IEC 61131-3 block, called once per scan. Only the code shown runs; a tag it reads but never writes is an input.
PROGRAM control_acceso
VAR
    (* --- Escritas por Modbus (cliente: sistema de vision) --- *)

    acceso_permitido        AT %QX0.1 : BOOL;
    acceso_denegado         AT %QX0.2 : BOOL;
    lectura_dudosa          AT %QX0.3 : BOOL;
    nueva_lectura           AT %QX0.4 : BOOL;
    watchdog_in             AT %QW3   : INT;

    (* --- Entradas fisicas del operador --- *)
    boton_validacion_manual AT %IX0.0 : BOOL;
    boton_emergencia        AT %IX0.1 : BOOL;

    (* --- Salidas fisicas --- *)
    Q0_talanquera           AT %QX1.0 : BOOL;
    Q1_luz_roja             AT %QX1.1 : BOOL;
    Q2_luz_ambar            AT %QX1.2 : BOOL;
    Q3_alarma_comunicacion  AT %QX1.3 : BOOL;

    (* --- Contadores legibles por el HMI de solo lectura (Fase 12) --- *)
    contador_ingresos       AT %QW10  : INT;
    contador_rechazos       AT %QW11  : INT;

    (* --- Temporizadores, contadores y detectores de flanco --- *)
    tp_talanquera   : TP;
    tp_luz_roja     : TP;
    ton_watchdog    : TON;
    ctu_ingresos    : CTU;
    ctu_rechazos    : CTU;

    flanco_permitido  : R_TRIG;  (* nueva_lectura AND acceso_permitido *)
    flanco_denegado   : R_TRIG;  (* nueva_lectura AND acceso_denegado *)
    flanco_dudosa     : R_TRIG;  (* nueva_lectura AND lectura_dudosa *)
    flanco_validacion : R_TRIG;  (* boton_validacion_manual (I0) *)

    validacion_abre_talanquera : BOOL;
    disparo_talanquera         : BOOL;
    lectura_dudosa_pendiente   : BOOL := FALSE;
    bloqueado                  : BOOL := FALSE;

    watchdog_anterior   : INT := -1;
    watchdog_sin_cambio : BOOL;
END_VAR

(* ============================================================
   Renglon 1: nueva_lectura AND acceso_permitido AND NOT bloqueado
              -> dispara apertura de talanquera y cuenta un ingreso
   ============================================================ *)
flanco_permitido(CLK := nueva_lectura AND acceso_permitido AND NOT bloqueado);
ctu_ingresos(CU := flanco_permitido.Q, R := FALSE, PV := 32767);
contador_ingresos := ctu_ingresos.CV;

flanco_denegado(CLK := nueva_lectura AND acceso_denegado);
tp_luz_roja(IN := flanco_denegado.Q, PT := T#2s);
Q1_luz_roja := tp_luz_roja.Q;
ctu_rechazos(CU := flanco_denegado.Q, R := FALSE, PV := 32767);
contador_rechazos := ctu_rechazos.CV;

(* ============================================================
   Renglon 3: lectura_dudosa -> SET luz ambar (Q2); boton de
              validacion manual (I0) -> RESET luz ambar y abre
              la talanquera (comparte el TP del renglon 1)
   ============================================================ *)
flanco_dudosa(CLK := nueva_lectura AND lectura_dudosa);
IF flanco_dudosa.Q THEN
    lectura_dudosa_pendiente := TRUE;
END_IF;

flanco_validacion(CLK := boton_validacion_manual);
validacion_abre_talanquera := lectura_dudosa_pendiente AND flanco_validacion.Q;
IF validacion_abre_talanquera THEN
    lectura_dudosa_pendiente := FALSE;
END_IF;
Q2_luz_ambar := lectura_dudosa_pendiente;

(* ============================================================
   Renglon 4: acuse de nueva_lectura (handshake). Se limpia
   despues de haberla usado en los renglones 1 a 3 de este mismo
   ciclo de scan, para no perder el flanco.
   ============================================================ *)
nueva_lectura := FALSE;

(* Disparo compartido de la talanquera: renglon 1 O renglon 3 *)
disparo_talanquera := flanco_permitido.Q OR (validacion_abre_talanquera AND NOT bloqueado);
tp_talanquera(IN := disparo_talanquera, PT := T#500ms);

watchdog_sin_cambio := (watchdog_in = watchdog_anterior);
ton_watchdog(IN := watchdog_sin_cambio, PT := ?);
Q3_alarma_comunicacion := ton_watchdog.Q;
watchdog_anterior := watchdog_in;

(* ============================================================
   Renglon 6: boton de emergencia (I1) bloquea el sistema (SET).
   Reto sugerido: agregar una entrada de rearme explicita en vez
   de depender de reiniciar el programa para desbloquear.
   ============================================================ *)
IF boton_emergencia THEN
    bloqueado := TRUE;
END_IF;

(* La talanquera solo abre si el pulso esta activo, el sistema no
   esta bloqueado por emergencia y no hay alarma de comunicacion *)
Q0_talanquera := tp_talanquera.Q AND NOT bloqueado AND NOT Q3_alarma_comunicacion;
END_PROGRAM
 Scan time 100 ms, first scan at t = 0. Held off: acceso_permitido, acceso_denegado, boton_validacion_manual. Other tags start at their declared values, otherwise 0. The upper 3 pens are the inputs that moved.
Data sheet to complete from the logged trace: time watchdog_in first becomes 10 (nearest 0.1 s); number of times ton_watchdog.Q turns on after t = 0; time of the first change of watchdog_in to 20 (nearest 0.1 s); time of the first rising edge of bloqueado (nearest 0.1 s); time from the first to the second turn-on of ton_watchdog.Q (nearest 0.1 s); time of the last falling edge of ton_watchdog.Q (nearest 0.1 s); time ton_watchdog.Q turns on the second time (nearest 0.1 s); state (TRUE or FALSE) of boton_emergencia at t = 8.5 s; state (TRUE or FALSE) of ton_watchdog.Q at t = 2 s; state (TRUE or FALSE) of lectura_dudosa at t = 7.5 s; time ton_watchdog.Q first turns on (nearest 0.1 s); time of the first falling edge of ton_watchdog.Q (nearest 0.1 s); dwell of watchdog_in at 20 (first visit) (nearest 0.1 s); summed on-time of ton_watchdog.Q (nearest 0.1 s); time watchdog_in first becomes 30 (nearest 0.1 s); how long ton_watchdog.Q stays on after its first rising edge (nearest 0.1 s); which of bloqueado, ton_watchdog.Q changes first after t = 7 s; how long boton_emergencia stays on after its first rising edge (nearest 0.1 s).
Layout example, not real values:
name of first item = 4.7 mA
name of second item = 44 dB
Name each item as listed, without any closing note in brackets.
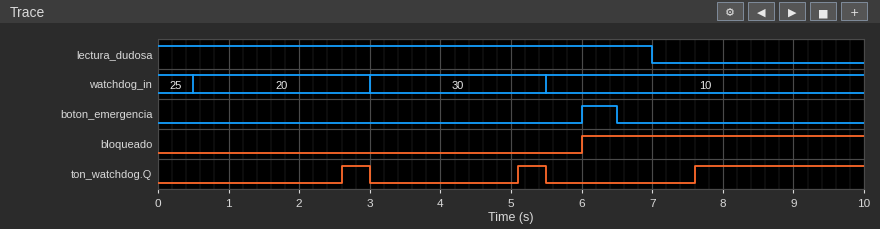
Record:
time watchdog_in first becomes 10 = 5.5 s
number of times ton_watchdog.Q turns on after t = 0 = 3
time of the first change of watchdog_in to 20 = 0.5 s
time of the first rising edge of bloqueado = 6.0 s
time from the first to the second turn-on of ton_watchdog.Q = 2.5 s
time of the last falling edge of ton_watchdog.Q = 5.5 s
time ton_watchdog.Q turns on the second time = 5.1 s
state (TRUE or FALSE) of boton_emergencia at t = 8.5 s = FALSE
state (TRUE or FALSE) of ton_watchdog.Q at t = 2 s = FALSE
state (TRUE or FALSE) of lectura_dudosa at t = 7.5 s = FALSE
time ton_watchdog.Q first turns on = 2.6 s
time of the first falling edge of ton_watchdog.Q = 3.0 s
dwell of watchdog_in at 20 (first visit) = 2.5 s
summed on-time of ton_watchdog.Q = 3.2 s
time watchdog_in first becomes 30 = 3.0 s
how long ton_watchdog.Q stays on after its first rising edge = 0.4 s
which of bloqueado, ton_watchdog.Q changes first after t = 7 s = ton_watchdog.Q
how long boton_emergencia stays on after its first rising edge = 0.5 s
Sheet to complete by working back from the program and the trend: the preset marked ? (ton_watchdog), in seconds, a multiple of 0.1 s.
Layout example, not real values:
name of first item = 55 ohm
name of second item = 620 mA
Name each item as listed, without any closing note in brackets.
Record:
the preset marked ? (ton_watchdog), in seconds, a multiple of 0.1 s = 2.0 s
